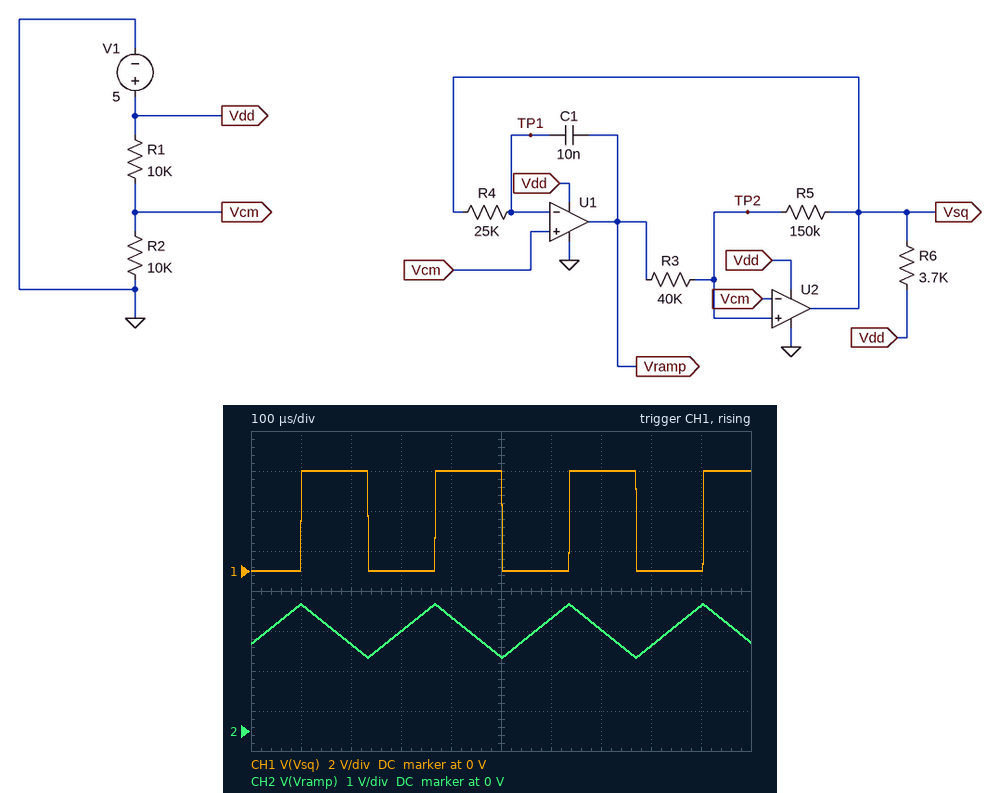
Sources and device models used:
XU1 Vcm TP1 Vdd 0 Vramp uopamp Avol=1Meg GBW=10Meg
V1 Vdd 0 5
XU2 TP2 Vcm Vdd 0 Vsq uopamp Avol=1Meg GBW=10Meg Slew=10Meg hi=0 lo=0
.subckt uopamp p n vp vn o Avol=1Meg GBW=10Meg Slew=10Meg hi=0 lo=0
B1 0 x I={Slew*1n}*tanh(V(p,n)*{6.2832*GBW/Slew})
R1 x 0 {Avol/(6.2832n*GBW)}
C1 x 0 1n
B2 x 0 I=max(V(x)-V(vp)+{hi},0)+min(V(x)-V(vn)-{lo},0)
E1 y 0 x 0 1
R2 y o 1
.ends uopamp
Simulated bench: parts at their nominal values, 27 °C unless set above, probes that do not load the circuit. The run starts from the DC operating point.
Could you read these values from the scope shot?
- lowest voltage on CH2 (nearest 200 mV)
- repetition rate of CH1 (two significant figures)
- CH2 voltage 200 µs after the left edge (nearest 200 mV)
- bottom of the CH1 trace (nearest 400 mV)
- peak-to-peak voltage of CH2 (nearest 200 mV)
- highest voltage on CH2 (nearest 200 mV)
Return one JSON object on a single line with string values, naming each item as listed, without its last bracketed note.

{"lowest voltage on CH2": "1.8 V", "repetition rate of CH1": "3.7 kHz", "CH2 voltage 200 µs after the left edge": "2.2 V", "bottom of the CH1 trace": "0 V", "peak-to-peak voltage of CH2": "1.4 V", "highest voltage on CH2": "3.2 V"}
